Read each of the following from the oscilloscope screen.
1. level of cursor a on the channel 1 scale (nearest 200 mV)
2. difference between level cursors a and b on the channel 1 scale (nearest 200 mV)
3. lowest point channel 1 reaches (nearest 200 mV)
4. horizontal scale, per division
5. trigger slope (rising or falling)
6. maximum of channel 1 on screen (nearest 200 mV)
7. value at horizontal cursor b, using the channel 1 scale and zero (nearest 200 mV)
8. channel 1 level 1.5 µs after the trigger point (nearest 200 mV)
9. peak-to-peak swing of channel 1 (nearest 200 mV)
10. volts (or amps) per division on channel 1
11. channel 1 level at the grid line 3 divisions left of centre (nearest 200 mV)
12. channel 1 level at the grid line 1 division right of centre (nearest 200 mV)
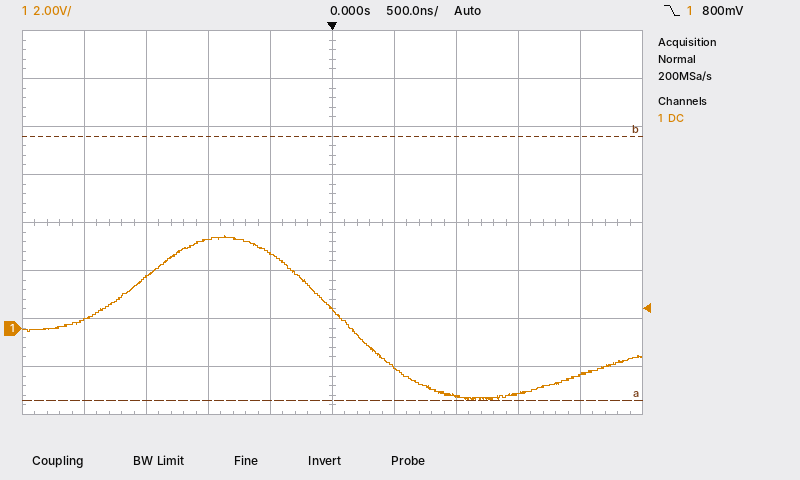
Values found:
-3.0 V
11.0 V
-3.0 V
500 ns
falling
3.8 V
8.0 V
-2.8 V
6.8 V
2 V
2.2 V
-1.6 V
